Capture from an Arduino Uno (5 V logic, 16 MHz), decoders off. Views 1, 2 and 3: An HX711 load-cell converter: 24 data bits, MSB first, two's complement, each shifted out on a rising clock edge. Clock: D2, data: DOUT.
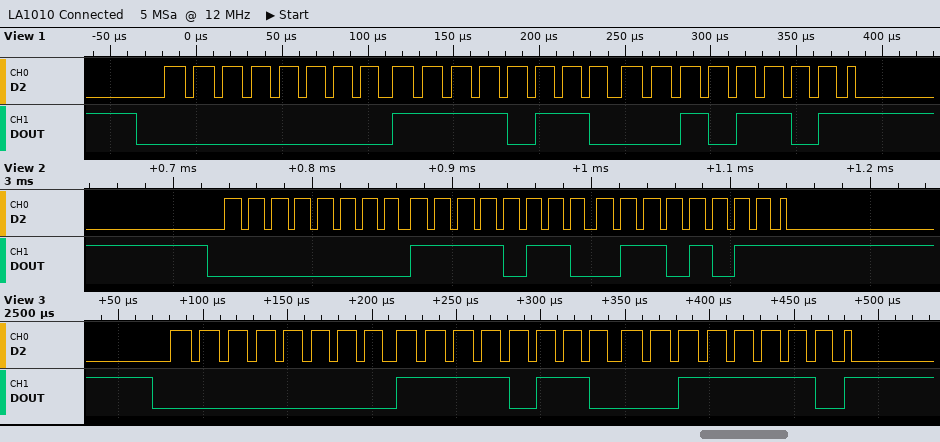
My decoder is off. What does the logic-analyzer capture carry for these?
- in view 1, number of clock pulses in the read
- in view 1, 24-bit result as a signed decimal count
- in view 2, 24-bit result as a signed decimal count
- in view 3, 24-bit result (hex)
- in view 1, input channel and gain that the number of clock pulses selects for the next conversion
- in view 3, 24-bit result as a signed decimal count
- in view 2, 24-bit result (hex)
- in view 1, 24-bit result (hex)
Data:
25
63021
63083
0x00F63E
channel A, gain 128
63038
0x00F66B
0x00F62D
